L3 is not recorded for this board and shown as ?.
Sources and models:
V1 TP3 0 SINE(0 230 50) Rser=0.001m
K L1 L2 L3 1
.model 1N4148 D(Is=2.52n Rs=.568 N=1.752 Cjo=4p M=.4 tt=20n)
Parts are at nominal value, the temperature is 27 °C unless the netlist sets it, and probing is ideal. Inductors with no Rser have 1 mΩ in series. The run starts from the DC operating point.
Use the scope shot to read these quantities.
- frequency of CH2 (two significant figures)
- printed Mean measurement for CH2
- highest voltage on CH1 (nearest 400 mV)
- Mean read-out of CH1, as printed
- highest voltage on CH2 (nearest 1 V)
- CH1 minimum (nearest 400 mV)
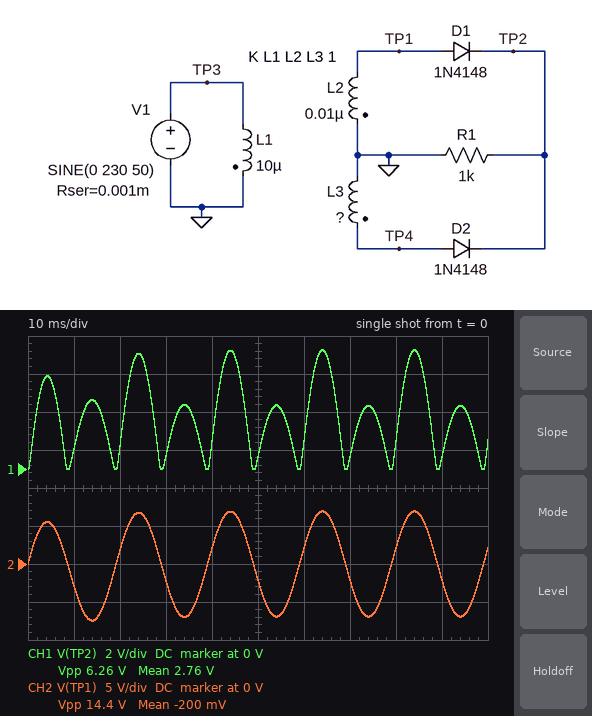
50 Hz
-200 mV
6.4 V
2.76 V
7 V
0 V
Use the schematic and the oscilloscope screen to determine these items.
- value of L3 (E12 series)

3.3 nH
